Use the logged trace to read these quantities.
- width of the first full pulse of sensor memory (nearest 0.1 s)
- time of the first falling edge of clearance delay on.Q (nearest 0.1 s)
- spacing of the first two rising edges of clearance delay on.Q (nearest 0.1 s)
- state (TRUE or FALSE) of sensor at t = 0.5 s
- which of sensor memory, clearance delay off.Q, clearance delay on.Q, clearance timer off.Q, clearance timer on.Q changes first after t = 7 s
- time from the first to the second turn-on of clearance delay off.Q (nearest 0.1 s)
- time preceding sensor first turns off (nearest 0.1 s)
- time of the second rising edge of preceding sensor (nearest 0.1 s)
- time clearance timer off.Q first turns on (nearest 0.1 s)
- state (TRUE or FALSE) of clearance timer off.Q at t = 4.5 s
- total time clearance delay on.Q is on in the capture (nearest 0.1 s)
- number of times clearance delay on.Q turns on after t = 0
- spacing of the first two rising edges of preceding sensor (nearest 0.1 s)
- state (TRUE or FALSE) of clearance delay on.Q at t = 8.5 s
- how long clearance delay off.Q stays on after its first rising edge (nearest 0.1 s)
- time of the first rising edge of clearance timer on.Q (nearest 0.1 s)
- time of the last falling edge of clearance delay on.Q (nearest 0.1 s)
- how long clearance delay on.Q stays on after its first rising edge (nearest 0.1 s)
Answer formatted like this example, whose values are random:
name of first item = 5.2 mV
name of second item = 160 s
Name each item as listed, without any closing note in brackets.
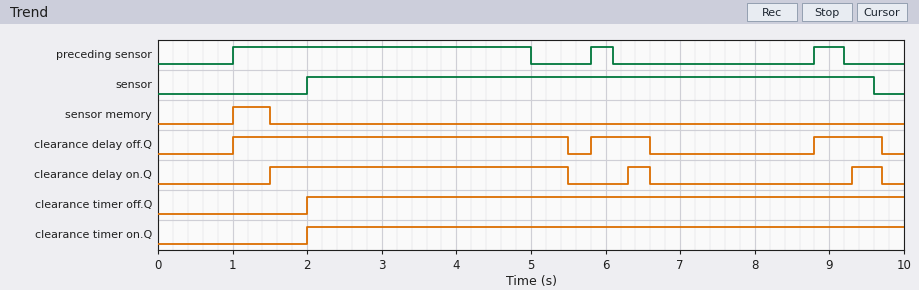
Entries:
width of the first full pulse of sensor memory = 0.5 s
time of the first falling edge of clearance delay on.Q = 5.5 s
spacing of the first two rising edges of clearance delay on.Q = 4.8 s
state (TRUE or FALSE) of sensor at t = 0.5 s = FALSE
which of sensor memory, clearance delay off.Q, clearance delay on.Q, clearance timer off.Q, clearance timer on.Q changes first after t = 7 s = clearance delay off.Q
time from the first to the second turn-on of clearance delay off.Q = 4.8 s
time preceding sensor first turns off = 5.0 s
time of the second rising edge of preceding sensor = 5.8 s
time clearance timer off.Q first turns on = 2.0 s
state (TRUE or FALSE) of clearance timer off.Q at t = 4.5 s = TRUE
total time clearance delay on.Q is on in the capture = 4.7 s
number of times clearance delay on.Q turns on after t = 0 = 3
spacing of the first two rising edges of preceding sensor = 4.8 s
state (TRUE or FALSE) of clearance delay on.Q at t = 8.5 s = FALSE
how long clearance delay off.Q stays on after its first rising edge = 4.5 s
time of the first rising edge of clearance timer on.Q = 2.0 s
time of the last falling edge of clearance delay on.Q = 9.7 s
how long clearance delay on.Q stays on after its first rising edge = 4.0 s
